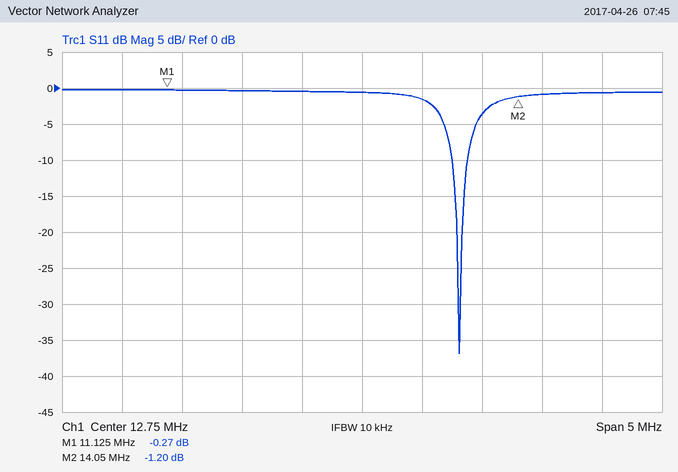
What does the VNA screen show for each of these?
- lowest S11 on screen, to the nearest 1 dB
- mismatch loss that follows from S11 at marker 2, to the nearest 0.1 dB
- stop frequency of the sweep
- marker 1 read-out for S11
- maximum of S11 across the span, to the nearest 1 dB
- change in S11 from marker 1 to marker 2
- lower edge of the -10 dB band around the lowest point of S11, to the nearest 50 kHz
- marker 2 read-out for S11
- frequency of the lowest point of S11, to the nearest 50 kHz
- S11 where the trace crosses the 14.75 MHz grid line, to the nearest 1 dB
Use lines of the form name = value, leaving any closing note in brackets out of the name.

lowest S11 on screen, to the nearest 1 dB = -37 dB
mismatch loss that follows from S11 at marker 2, to the nearest 0.1 dB = 6.2 dB
stop frequency of the sweep = 15.25 MHz
marker 1 read-out for S11 = -0.27 dB
maximum of S11 across the span, to the nearest 1 dB = 0 dB
change in S11 from marker 1 to marker 2 = -0.93 dB
lower edge of the -10 dB band around the lowest point of S11, to the nearest 50 kHz = 13.50 MHz
marker 2 read-out for S11 = -1.20 dB
frequency of the lowest point of S11, to the nearest 50 kHz = 13.55 MHz
S11 where the trace crosses the 14.75 MHz grid line, to the nearest 1 dB = -1 dB
